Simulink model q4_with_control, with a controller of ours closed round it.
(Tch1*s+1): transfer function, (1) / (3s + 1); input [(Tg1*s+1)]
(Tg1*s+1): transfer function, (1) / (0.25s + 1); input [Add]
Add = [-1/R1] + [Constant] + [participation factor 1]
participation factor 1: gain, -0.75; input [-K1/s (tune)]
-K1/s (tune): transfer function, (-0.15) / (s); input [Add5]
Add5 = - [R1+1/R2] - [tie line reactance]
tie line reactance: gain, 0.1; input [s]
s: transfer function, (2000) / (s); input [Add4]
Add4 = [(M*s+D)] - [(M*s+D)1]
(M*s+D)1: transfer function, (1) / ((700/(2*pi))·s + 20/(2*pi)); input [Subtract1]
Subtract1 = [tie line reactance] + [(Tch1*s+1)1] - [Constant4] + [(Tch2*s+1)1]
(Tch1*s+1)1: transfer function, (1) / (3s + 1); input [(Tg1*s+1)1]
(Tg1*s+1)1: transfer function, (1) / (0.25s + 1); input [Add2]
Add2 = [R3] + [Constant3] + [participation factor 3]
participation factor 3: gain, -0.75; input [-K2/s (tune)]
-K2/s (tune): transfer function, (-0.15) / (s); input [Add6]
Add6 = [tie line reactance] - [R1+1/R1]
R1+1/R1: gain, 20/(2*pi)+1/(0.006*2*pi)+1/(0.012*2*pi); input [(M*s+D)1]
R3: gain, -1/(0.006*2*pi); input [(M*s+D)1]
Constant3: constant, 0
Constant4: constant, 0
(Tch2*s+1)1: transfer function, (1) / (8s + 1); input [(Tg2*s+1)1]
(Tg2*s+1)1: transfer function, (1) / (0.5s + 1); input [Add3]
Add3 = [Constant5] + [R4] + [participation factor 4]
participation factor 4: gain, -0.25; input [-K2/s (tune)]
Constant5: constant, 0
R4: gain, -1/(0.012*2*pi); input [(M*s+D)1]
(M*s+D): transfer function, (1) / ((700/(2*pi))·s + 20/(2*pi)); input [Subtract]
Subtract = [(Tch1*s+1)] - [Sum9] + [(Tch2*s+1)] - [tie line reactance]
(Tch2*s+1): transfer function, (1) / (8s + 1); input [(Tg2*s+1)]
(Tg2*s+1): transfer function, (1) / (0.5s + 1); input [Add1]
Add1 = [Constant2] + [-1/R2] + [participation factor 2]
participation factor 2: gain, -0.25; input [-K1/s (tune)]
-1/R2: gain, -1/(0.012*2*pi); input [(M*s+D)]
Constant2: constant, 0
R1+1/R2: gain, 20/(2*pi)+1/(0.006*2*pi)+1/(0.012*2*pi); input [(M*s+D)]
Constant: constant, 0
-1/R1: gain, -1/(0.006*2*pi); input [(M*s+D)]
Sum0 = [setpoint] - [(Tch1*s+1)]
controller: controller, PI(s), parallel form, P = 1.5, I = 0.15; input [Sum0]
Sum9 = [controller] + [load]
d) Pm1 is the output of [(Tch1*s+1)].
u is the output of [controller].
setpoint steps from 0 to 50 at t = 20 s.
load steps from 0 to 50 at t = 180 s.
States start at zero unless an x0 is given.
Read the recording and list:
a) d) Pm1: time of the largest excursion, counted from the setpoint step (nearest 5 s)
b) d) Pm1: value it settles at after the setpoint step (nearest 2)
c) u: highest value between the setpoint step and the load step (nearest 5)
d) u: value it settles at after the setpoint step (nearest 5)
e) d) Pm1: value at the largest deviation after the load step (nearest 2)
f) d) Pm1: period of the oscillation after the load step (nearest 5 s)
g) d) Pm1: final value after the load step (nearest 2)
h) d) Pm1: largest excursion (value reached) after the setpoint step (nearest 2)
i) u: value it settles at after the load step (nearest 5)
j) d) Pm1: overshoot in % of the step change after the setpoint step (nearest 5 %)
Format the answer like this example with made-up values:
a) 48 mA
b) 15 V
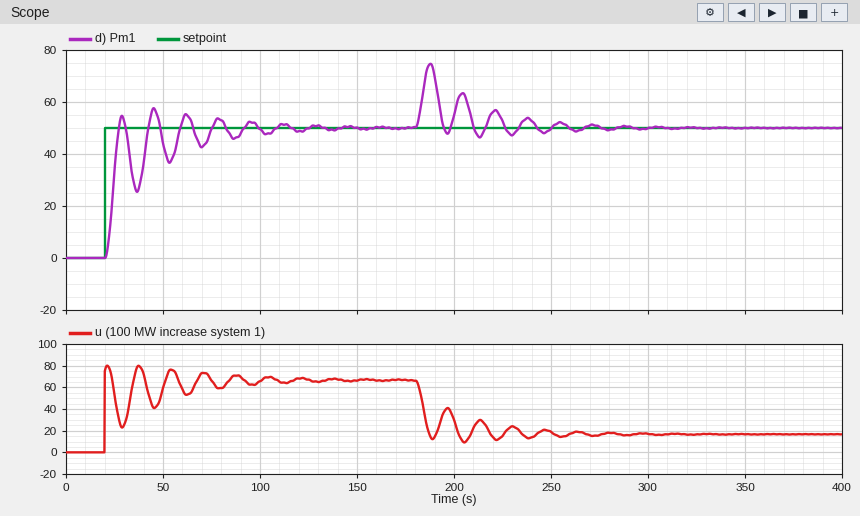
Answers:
a) 25 s
b) 50
c) 80
d) 65
e) 74
f) 15 s
g) 50
h) 58
i) 15
j) 15 %
